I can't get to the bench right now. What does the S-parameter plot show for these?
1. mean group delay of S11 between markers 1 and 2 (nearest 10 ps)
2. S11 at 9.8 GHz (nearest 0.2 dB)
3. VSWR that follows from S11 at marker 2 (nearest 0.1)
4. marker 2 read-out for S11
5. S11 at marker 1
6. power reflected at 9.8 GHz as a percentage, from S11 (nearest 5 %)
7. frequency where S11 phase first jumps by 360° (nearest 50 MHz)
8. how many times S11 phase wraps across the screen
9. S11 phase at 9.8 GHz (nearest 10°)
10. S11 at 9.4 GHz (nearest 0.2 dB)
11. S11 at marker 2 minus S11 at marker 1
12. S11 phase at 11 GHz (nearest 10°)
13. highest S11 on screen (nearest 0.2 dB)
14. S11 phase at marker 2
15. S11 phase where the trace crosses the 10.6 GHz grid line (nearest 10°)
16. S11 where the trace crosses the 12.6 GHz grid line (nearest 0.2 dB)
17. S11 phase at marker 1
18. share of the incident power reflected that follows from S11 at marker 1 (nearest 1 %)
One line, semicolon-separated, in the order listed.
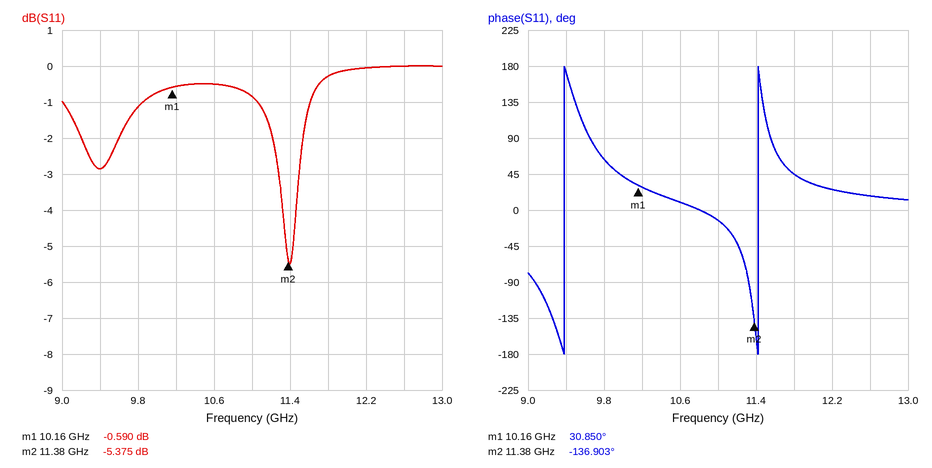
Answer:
380 ps; -1.2 dB; 3.3; -5.375 dB; -0.590 dB; 75 %; 9.40 GHz; 2; 60°; -2.8 dB; -4.785 dB; -10°; 0.0 dB; -136.903°; 10°; 0.0 dB; 30.850°; 87 %
